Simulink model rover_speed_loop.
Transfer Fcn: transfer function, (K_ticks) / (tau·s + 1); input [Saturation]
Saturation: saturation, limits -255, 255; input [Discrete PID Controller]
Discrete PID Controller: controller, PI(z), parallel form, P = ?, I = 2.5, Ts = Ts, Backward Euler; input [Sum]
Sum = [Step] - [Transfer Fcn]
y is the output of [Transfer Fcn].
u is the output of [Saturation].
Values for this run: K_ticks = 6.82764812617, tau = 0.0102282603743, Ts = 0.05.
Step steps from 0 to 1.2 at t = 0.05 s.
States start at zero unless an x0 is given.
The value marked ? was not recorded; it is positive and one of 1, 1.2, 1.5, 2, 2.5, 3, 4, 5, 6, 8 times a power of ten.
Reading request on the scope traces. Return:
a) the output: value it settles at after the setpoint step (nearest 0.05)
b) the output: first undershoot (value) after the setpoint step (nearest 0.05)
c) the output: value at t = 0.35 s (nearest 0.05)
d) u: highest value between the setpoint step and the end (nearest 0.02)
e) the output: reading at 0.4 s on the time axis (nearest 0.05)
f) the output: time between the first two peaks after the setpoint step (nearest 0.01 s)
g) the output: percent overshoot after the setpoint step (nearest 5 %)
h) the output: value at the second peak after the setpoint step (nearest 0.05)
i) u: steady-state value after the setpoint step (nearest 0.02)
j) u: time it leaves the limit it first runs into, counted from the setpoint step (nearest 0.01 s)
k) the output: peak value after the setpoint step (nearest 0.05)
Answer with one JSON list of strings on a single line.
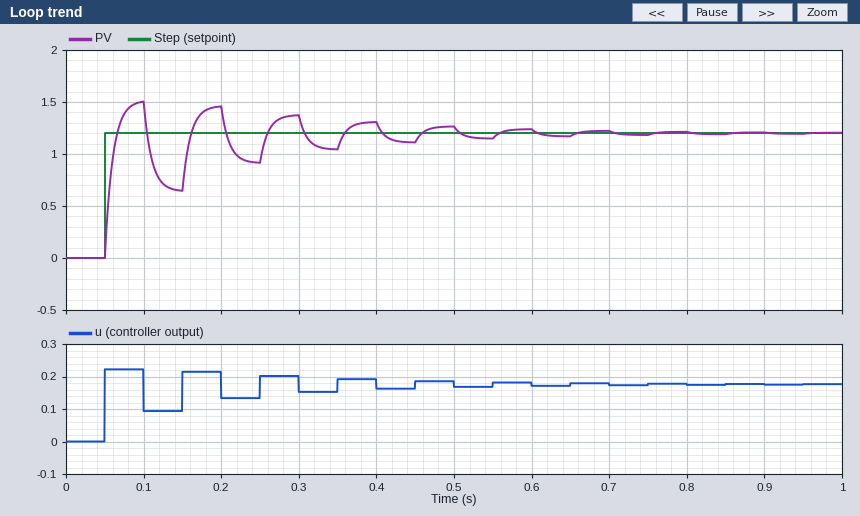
["1.20", "0.65", "1.05", "0.22", "1.30", "0.10 s", "25 %", "1.45", "0.18", "0.05 s", "1.50"]
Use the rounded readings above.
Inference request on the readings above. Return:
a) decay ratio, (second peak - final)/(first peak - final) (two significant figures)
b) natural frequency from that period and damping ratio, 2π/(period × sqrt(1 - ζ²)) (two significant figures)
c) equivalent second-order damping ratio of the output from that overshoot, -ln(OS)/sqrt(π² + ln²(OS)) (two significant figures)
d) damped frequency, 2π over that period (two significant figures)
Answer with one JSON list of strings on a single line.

["0.83", "69 rad/s", "0.40", "63 rad/s"]
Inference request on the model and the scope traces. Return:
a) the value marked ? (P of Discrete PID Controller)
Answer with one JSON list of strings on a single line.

["0.06"]
